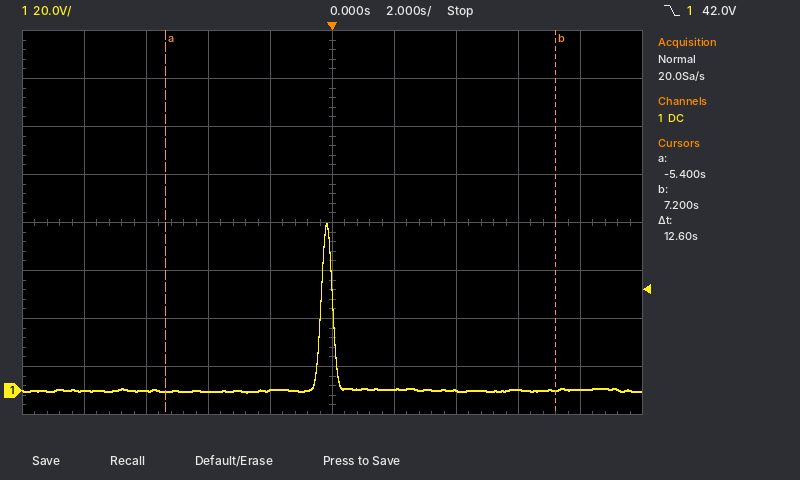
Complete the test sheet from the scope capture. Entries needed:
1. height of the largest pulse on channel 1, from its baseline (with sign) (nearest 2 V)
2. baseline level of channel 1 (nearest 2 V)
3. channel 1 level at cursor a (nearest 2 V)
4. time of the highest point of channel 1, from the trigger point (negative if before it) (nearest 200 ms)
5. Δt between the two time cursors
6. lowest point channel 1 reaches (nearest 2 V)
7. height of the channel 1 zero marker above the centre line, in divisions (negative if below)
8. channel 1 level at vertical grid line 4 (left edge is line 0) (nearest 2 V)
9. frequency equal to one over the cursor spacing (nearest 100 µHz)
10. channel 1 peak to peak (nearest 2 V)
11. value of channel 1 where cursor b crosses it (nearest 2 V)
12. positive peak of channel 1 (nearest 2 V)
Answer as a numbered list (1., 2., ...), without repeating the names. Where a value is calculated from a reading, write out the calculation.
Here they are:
1. 70 V − (0 V) = +70 V
2. 0 V
3. 0 V
4. -200 ms
5. 12.6 s
6. 0 V
7. -3.5 div
8. 0 V
9. 1 / 12.6 s ≈ 79.4 mHz
10. 70 V − (0 V) = 70 V
11. 0 V
12. 70 V
